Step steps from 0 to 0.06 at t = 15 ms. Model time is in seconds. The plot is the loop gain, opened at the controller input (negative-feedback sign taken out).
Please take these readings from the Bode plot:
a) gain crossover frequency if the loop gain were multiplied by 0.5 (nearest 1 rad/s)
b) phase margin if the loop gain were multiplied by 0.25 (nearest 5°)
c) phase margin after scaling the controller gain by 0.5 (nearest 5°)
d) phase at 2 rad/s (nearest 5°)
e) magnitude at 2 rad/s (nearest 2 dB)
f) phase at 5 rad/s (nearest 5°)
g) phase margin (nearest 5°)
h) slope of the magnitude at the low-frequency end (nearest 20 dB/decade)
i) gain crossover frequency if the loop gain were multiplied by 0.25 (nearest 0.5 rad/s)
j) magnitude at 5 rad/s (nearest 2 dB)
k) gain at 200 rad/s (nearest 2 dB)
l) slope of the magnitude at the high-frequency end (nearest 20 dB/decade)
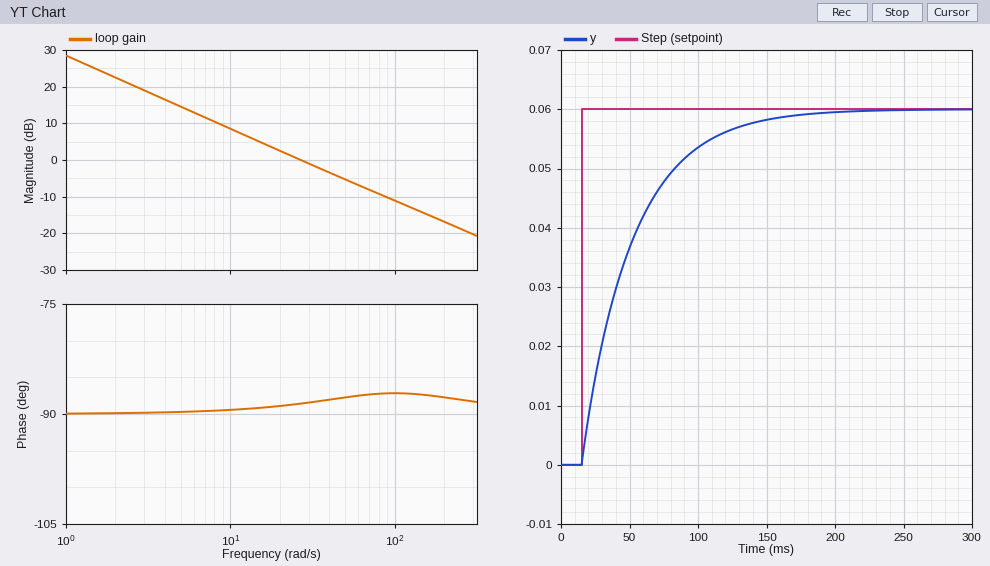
13 rad/s
90°
90°
-90°
22 dB
-90°
90°
-20 dB/decade
6.5 rad/s
14 dB
-16 dB
-20 dB/decade
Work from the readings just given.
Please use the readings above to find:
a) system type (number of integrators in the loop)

1
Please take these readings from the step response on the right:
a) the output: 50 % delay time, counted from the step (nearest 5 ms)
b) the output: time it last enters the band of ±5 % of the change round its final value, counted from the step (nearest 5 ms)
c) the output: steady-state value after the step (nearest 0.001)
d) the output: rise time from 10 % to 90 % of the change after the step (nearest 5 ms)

25 ms
115 ms
0.060
85 ms
